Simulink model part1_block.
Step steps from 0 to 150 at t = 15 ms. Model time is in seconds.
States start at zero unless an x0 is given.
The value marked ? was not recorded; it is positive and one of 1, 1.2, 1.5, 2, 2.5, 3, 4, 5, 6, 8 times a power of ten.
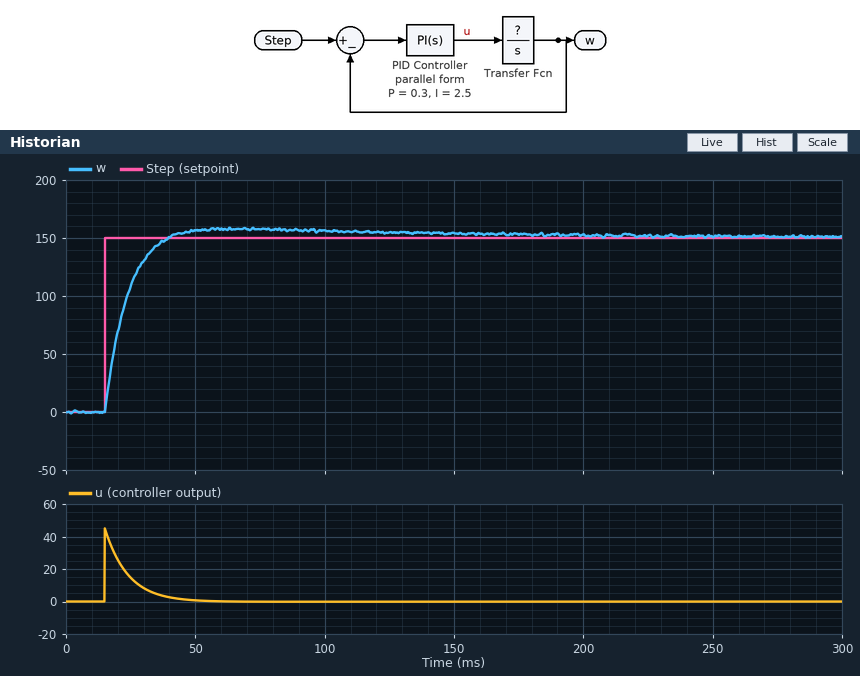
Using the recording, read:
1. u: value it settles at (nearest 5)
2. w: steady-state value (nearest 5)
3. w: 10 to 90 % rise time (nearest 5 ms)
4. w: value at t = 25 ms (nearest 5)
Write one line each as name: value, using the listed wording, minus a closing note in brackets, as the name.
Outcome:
u: value it settles at: 0
w: steady-state value: 150
w: 10 to 90 % rise time: 15 ms
w: value at t = 25 ms: 110
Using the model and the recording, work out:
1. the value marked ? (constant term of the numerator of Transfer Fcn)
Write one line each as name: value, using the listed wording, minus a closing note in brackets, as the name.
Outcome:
the value marked ?: 400
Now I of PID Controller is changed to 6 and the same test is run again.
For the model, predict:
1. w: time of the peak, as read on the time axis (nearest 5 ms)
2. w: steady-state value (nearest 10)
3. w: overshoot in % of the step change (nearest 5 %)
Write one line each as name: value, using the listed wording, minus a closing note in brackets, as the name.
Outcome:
w: time of the peak, as read on the time axis: 55 ms
w: steady-state value: 150
w: overshoot in % of the step change: 10 %
